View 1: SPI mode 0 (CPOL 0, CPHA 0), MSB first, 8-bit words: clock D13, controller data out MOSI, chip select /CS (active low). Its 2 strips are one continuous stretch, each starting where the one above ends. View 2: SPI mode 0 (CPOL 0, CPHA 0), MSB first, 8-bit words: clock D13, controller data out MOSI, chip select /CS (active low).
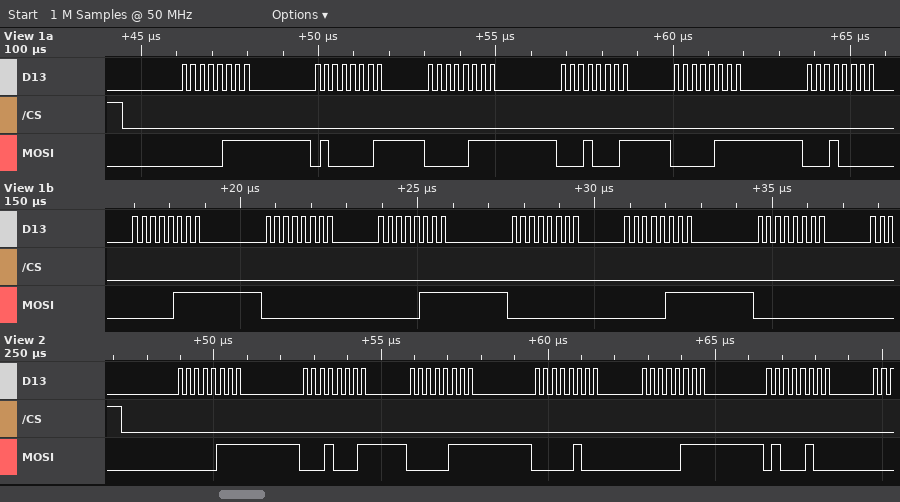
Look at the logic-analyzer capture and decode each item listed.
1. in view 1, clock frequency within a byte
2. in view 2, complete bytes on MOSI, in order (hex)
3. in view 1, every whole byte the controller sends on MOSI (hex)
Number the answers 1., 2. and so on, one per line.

1. 4 MHz
2. 07 11 07 04 07 44
3. 07 41 07 11 07 10 07 00 07 00 07 00
